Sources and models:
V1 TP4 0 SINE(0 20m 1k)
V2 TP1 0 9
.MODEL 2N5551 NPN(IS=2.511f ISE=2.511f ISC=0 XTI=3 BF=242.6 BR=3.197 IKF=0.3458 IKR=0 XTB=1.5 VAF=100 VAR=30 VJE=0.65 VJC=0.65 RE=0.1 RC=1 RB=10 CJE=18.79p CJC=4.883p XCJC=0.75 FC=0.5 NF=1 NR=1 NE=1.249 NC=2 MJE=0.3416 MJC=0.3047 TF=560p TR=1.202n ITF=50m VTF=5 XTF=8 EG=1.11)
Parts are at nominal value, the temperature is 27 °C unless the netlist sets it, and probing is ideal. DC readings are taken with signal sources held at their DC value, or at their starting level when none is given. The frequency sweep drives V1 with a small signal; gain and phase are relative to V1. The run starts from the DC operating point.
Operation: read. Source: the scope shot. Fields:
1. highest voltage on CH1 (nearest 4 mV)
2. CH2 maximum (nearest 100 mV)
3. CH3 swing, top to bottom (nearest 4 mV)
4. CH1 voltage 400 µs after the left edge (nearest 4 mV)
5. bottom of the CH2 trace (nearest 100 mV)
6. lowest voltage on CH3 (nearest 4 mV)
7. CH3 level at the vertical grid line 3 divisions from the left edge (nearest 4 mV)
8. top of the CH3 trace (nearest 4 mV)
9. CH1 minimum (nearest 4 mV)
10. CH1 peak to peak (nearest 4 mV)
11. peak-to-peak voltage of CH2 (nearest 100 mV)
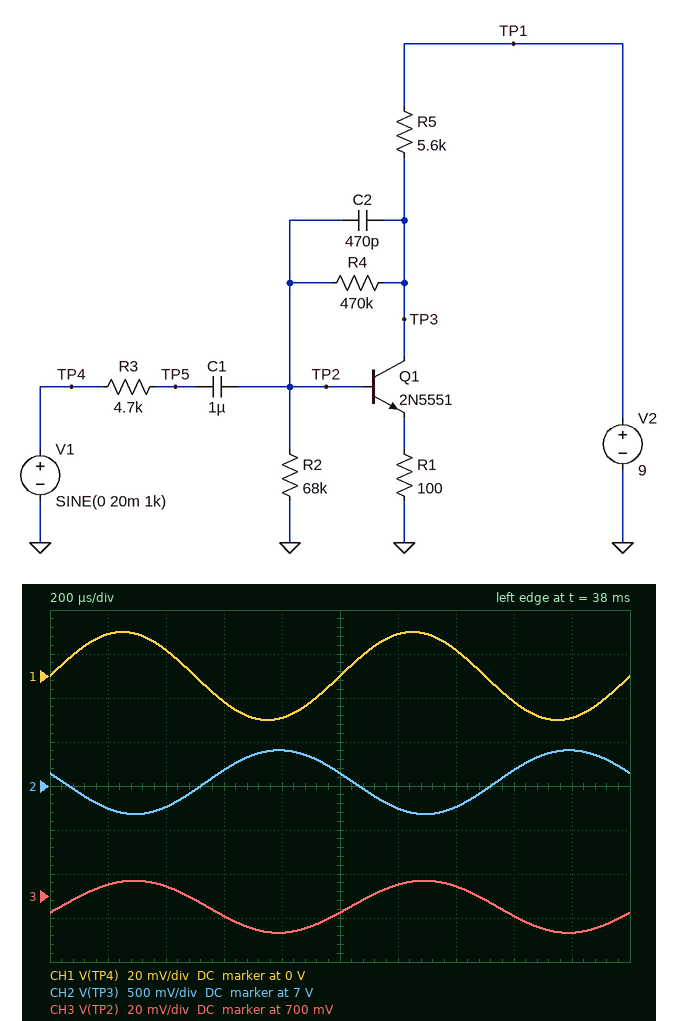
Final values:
20 mV
7.4 V
24 mV
12 mV
6.7 V
684 mV
692 mV
708 mV
-20 mV
40 mV
700 mV
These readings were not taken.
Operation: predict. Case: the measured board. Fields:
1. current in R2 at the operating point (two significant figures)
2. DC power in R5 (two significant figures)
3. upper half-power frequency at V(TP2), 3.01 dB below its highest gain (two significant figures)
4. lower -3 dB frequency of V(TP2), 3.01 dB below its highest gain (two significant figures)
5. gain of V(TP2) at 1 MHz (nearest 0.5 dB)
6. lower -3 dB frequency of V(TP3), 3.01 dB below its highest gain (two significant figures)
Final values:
10 µA
680 µW
3.5 kHz
13 Hz
-29.0 dB
13 Hz
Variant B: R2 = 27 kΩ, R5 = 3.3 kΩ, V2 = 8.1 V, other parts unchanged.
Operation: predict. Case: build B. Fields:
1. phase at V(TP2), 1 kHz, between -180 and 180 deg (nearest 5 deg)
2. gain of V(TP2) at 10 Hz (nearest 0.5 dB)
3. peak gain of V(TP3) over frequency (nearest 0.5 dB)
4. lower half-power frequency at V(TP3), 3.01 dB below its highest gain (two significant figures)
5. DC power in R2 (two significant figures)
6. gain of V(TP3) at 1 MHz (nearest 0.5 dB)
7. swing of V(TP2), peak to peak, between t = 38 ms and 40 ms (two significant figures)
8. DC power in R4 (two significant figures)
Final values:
0 deg
-2.5 dB
-8.5 dB
45 kHz
7.1 µW
-9.0 dB
34 mV
120 µW
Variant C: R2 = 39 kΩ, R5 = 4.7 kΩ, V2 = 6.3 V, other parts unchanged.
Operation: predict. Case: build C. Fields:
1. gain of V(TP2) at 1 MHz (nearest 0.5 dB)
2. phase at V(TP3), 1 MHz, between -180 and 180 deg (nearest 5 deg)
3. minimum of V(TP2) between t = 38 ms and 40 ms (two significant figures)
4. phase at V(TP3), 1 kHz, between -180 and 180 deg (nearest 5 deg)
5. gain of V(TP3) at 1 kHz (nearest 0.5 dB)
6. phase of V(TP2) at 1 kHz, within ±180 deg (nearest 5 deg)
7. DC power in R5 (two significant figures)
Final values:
-7.5 dB
-20 deg
460 mV
160 deg
-28.5 dB
0 deg
740 nW
